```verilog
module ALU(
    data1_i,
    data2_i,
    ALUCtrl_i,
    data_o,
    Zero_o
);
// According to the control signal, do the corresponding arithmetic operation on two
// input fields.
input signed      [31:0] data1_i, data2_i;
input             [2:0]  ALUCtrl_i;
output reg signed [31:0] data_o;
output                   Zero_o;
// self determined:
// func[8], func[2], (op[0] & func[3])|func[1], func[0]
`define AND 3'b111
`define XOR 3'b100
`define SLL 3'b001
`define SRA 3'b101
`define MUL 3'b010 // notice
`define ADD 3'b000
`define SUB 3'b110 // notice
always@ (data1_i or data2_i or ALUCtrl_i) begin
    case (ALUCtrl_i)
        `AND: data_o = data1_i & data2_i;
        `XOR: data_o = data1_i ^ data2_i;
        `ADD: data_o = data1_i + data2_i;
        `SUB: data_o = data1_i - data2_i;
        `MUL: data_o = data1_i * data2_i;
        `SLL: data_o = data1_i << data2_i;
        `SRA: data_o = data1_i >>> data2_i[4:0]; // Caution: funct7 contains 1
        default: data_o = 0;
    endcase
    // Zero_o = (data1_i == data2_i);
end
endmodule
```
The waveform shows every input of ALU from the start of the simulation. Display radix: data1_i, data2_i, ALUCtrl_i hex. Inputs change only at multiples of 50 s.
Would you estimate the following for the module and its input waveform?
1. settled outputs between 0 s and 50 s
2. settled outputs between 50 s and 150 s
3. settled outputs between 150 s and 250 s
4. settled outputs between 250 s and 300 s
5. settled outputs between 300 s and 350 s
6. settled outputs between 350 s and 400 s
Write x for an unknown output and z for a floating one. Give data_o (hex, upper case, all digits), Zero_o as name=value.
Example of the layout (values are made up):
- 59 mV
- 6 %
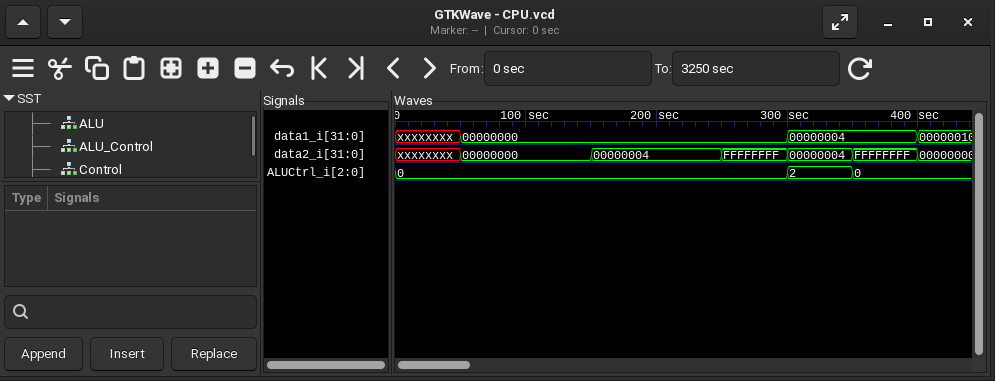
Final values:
- data_o=x, Zero_o=z
- data_o=00000000, Zero_o=z
- data_o=00000004, Zero_o=z
- data_o=FFFFFFFF, Zero_o=z
- data_o=00000010, Zero_o=z
- data_o=00000003, Zero_o=z
